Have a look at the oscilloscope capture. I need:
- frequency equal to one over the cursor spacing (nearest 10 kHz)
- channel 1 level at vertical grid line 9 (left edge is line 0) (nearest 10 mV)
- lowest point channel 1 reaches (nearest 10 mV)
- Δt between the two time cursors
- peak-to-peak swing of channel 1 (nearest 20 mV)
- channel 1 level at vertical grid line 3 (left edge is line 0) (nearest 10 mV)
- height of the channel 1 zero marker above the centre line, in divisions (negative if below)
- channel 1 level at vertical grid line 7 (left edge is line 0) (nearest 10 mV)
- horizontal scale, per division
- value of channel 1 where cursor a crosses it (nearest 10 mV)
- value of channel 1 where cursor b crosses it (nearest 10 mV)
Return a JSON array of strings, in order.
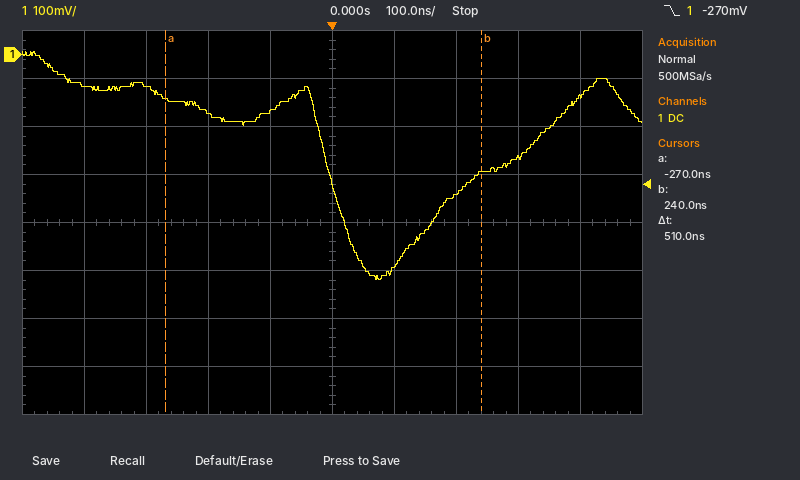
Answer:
["1.96 MHz", "-90 mV", "-470 mV", "510 ns", "480 mV", "-120 mV", "+3.5 div", "-290 mV", "100 ns", "-90 mV", "-250 mV"]
